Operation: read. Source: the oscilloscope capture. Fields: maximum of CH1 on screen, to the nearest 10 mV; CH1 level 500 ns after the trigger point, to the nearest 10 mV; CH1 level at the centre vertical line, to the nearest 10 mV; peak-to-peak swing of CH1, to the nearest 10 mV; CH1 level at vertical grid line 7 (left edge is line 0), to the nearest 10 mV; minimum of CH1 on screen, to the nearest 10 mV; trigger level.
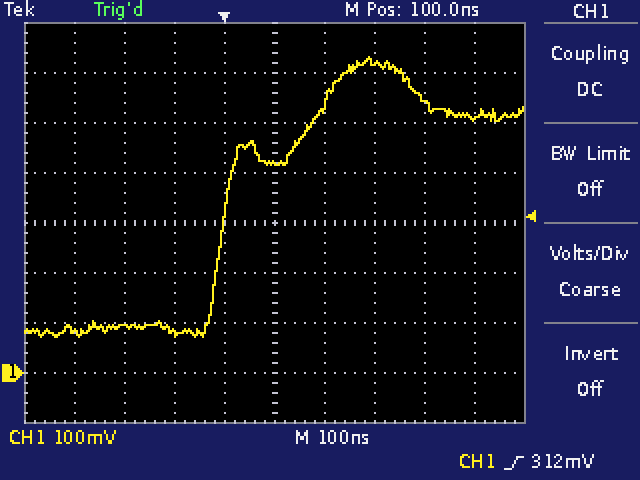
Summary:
630 mV
510 mV
420 mV
560 mV
620 mV
70 mV
312 mV
